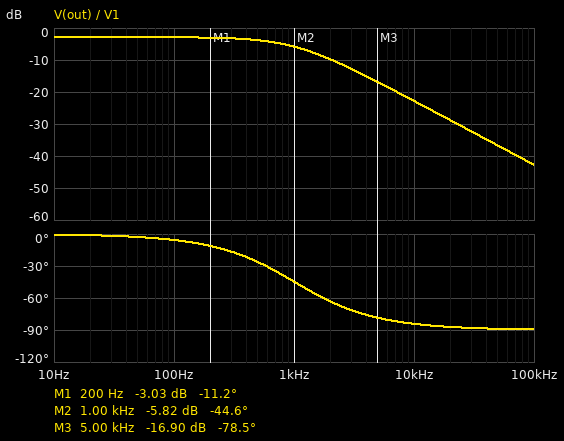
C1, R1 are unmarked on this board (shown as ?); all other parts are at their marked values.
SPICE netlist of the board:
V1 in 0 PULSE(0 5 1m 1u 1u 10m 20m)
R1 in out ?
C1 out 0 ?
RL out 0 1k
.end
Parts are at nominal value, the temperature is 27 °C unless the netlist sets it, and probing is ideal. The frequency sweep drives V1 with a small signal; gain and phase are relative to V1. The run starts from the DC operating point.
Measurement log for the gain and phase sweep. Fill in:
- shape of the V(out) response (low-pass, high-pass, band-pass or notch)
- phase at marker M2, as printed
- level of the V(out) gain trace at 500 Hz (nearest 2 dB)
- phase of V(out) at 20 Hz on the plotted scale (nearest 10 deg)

low-pass
-44.6 deg
-4 dB
0 deg
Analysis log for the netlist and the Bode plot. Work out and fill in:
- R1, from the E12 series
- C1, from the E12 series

390 Ω
560 nF
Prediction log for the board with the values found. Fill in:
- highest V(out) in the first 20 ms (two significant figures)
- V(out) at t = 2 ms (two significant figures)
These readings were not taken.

3.6 V
3.6 V
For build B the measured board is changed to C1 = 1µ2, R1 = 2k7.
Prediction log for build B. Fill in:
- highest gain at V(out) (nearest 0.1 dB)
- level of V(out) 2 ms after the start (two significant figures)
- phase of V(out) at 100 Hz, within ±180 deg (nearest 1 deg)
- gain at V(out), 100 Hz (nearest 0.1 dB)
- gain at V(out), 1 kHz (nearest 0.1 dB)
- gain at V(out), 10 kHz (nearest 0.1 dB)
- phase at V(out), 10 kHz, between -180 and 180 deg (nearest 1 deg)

-11.4 dB
920 mV
-29 deg
-12.5 dB
-26.3 dB
-46.2 dB
-89 deg
